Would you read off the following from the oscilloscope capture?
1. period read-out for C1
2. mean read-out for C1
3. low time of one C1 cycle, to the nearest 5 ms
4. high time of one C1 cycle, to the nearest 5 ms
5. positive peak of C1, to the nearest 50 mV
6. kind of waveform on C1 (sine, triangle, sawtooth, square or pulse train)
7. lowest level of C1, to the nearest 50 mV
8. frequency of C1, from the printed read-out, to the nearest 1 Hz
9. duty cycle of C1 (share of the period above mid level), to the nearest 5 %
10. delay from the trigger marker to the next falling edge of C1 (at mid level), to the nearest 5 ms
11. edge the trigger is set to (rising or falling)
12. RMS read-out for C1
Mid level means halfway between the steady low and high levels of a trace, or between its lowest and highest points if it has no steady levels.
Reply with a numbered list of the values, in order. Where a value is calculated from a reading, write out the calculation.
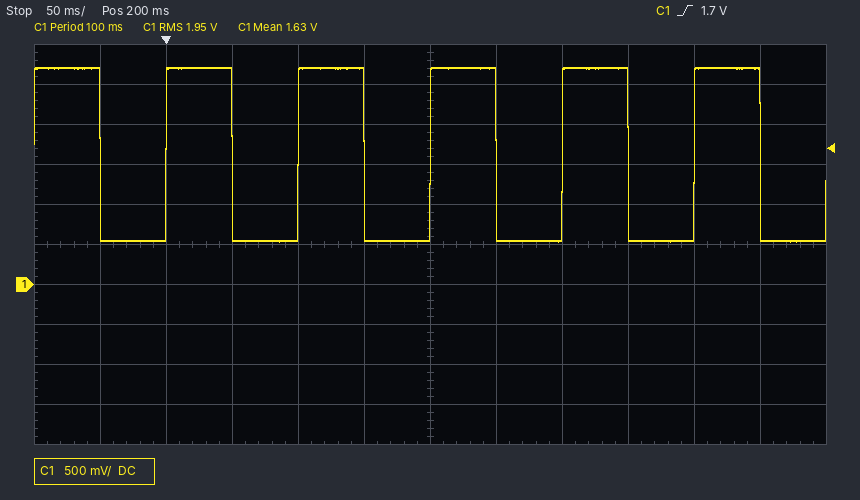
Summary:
1. 100 ms
2. 1.63 V
3. 50 ms
4. 50 ms
5. 2.70 V
6. square
7. 550 mV
8. 1 / 100 ms ≈ 10 Hz
9. 50 %
10. 50 ms
11. rising
12. 1.95 V
